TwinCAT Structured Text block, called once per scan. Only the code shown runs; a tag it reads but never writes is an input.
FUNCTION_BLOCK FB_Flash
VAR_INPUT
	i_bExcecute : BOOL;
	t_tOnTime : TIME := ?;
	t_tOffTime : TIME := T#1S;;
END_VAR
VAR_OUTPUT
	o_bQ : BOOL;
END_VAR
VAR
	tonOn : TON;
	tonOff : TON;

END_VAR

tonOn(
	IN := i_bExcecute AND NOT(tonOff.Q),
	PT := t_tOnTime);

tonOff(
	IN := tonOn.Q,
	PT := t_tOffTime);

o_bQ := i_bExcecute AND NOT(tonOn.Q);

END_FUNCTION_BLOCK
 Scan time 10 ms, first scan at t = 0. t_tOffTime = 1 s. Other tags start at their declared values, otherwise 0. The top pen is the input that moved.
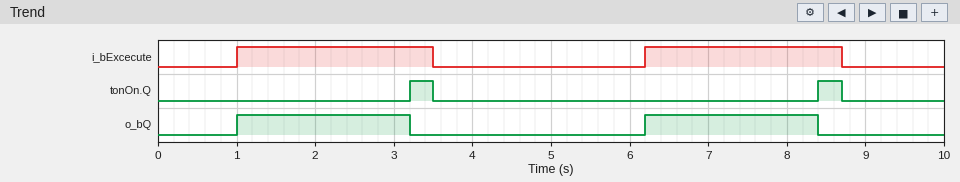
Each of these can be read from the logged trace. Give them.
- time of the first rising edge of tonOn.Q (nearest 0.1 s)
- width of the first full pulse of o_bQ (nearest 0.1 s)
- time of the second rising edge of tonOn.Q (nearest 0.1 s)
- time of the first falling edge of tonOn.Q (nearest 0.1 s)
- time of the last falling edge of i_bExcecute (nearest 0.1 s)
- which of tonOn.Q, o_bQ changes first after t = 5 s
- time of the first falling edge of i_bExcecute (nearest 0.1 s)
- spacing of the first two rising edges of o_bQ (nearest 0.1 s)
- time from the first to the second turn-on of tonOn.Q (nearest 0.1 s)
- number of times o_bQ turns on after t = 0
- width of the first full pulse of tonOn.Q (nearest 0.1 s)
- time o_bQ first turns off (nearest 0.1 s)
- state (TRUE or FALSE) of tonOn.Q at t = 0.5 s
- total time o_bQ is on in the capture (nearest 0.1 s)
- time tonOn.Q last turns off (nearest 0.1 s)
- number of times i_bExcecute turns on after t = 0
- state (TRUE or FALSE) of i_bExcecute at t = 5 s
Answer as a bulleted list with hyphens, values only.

- 3.2 s
- 2.2 s
- 8.4 s
- 3.5 s
- 8.7 s
- o_bQ
- 3.5 s
- 5.2 s
- 5.2 s
- 2
- 0.3 s
- 3.2 s
- FALSE
- 4.4 s
- 8.7 s
- 2
- FALSE
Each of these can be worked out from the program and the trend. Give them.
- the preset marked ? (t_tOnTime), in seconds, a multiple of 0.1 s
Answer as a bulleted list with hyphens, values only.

- 2.2 s
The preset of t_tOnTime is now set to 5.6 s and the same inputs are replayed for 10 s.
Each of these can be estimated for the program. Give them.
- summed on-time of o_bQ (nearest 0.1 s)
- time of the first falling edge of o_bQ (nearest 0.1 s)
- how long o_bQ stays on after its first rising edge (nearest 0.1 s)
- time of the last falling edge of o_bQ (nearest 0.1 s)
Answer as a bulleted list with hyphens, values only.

- 5.0 s
- 3.5 s
- 2.5 s
- 8.7 s
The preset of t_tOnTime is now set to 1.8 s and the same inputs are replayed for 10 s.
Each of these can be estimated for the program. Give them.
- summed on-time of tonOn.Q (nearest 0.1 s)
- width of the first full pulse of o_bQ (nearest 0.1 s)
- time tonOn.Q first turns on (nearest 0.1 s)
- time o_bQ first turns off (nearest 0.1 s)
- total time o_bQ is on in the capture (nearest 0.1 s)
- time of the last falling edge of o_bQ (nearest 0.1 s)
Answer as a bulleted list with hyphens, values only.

- 1.4 s
- 1.8 s
- 2.8 s
- 2.8 s
- 3.6 s
- 8.0 s
